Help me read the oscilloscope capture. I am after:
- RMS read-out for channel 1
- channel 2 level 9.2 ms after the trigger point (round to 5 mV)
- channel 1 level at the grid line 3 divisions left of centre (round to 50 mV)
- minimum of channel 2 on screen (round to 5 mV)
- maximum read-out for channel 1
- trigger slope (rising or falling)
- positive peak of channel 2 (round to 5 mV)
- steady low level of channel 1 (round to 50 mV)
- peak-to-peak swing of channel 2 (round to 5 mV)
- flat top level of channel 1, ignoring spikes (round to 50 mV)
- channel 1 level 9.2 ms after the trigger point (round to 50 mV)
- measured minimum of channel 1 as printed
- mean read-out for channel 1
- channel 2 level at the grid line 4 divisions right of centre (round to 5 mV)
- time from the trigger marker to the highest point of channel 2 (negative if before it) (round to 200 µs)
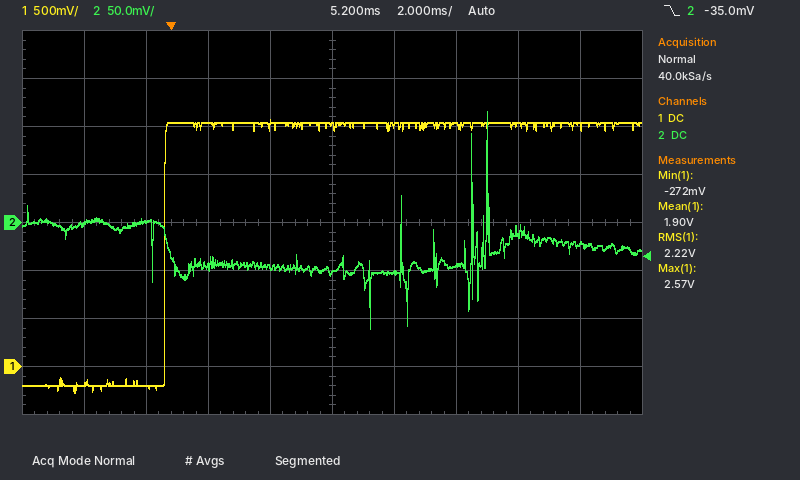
2.22 V
-45 mV
-200 mV
-110 mV
2.57 V
falling
115 mV
-200 mV
225 mV
2.55 V
2.50 V
-272 mV
1.90 V
-20 mV
+10.2 ms
